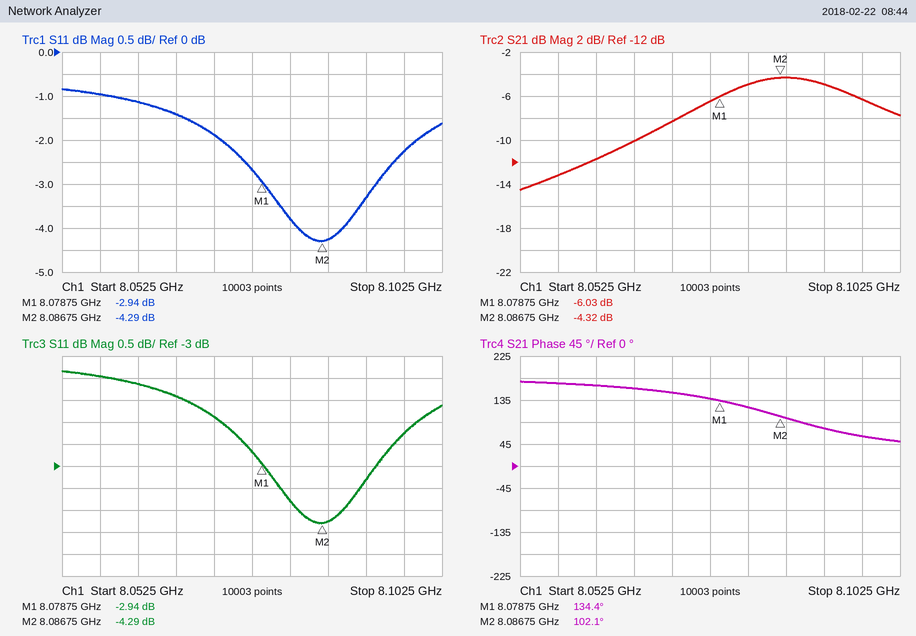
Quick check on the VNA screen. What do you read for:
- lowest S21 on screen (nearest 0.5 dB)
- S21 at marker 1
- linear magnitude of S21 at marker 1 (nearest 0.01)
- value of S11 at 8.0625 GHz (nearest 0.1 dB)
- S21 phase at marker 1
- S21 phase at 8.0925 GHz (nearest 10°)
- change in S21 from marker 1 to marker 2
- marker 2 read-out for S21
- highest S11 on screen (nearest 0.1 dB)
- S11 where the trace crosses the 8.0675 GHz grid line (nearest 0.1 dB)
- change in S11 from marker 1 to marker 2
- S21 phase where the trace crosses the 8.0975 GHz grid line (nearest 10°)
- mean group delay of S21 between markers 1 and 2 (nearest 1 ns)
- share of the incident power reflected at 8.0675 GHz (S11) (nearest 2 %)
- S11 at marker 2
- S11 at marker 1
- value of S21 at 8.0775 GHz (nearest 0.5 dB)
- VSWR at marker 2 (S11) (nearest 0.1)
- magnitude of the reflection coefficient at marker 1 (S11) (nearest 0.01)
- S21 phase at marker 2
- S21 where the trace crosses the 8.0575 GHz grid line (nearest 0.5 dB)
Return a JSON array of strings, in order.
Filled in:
["-14.5 dB", "-6.03 dB", "0.50", "-1.1 dB", "134.4°", "80°", "1.71 dB", "-4.32 dB", "-0.8 dB", "-1.4 dB", "-1.35 dB", "60°", "11 ns", "72 %", "-4.29 dB", "-2.94 dB", "-6.5 dB", "4.1", "0.71", "102.1°", "-13.0 dB"]
